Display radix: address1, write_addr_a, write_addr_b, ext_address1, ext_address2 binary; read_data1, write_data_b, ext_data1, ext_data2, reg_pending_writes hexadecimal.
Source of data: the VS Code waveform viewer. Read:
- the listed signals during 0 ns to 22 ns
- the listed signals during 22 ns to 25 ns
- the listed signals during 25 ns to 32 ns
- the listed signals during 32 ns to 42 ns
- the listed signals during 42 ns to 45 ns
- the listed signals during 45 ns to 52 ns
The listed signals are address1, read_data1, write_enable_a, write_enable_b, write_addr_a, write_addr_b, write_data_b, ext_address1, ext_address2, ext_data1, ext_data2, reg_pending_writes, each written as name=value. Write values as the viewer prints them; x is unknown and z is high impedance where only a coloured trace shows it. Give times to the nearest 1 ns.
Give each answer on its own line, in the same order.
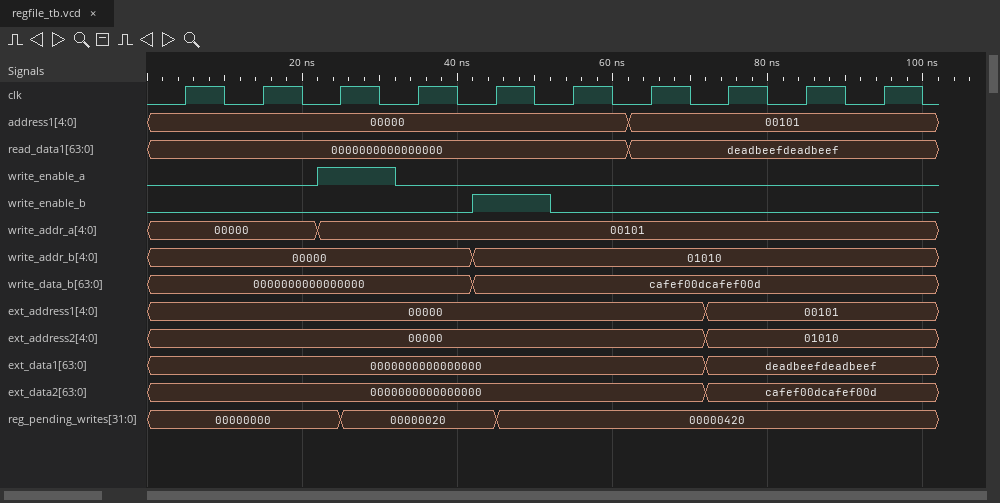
address1=00000, read_data1=0000000000000000, write_enable_a=0, write_enable_b=0, write_addr_a=00000, write_addr_b=00000, write_data_b=0000000000000000, ext_address1=00000, ext_address2=00000, ext_data1=0000000000000000, ext_data2=0000000000000000, reg_pending_writes=00000000
address1=00000, read_data1=0000000000000000, write_enable_a=1, write_enable_b=0, write_addr_a=00101, write_addr_b=00000, write_data_b=0000000000000000, ext_address1=00000, ext_address2=00000, ext_data1=0000000000000000, ext_data2=0000000000000000, reg_pending_writes=00000000
address1=00000, read_data1=0000000000000000, write_enable_a=1, write_enable_b=0, write_addr_a=00101, write_addr_b=00000, write_data_b=0000000000000000, ext_address1=00000, ext_address2=00000, ext_data1=0000000000000000, ext_data2=0000000000000000, reg_pending_writes=00000020
address1=00000, read_data1=0000000000000000, write_enable_a=0, write_enable_b=0, write_addr_a=00101, write_addr_b=00000, write_data_b=0000000000000000, ext_address1=00000, ext_address2=00000, ext_data1=0000000000000000, ext_data2=0000000000000000, reg_pending_writes=00000020
address1=00000, read_data1=0000000000000000, write_enable_a=0, write_enable_b=1, write_addr_a=00101, write_addr_b=01010, write_data_b=cafef00dcafef00d, ext_address1=00000, ext_address2=00000, ext_data1=0000000000000000, ext_data2=0000000000000000, reg_pending_writes=00000020
address1=00000, read_data1=0000000000000000, write_enable_a=0, write_enable_b=1, write_addr_a=00101, write_addr_b=01010, write_data_b=cafef00dcafef00d, ext_address1=00000, ext_address2=00000, ext_data1=0000000000000000, ext_data2=0000000000000000, reg_pending_writes=00000420
